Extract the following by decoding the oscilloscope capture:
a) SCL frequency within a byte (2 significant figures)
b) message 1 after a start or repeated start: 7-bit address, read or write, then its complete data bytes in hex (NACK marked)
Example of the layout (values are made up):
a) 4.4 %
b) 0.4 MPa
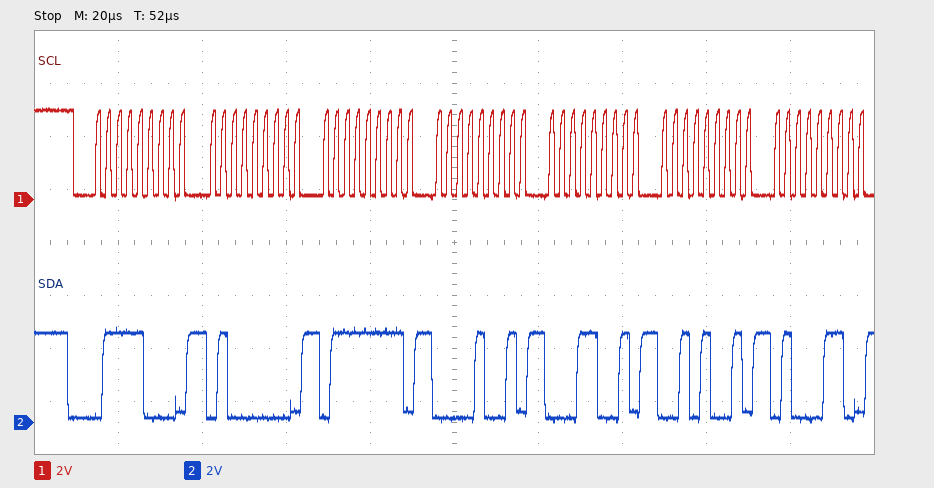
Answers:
a) 400 kHz
b) 0x3C write: 40 7F 09 19 29 46
